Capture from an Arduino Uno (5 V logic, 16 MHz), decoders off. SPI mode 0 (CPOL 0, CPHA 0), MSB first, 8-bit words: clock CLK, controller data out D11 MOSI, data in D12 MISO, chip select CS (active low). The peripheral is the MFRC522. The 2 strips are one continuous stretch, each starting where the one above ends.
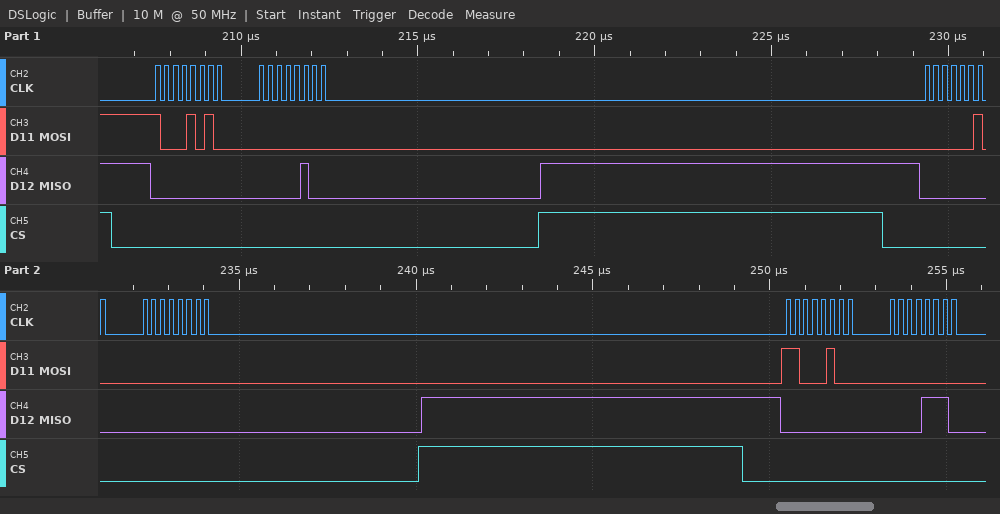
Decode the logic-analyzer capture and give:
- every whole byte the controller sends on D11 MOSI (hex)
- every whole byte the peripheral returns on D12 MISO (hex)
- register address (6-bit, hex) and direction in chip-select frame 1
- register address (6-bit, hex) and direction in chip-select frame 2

8A 00 02 00 C4 00
00 04 00 00 00 0E
0x05 read
0x01 write
